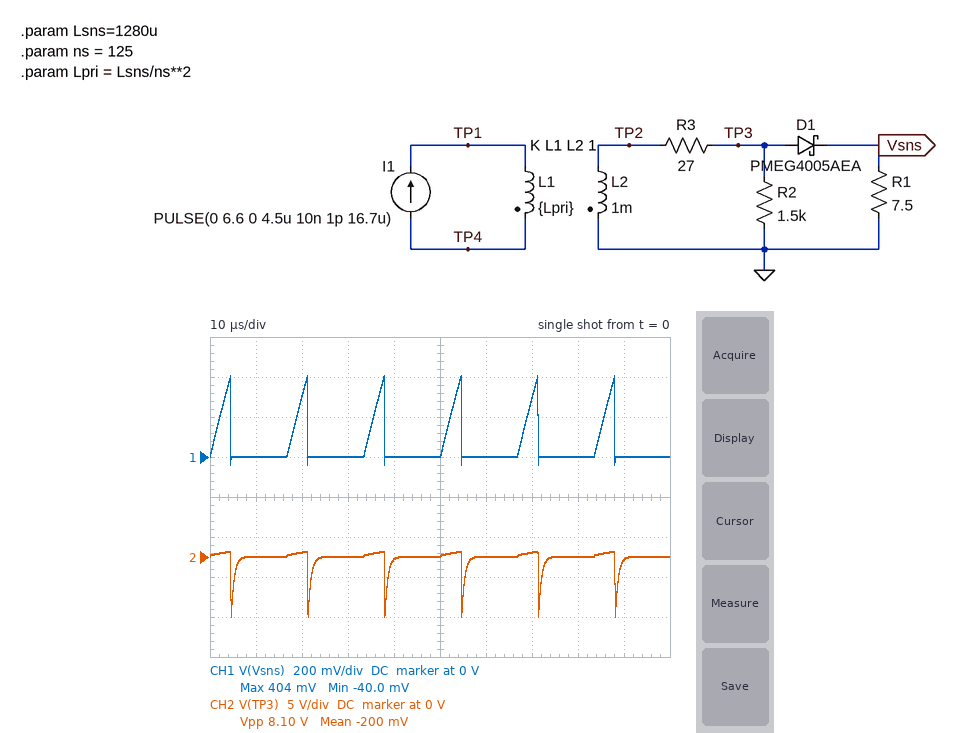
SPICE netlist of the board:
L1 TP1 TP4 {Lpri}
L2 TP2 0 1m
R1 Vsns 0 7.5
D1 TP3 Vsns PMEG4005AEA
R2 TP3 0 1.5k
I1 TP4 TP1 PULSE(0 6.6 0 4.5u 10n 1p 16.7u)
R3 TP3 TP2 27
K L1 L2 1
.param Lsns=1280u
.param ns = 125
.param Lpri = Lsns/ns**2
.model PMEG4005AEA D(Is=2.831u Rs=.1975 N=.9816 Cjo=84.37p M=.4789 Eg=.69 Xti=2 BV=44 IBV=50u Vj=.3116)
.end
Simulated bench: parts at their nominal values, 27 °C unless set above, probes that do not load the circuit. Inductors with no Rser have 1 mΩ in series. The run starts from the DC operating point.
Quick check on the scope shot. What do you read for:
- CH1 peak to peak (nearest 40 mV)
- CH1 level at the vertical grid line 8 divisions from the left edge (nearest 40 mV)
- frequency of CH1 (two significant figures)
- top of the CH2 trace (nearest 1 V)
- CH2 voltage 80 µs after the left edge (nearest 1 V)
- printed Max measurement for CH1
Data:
440 mV
0 V
60 kHz
1 V
0 V
404 mV
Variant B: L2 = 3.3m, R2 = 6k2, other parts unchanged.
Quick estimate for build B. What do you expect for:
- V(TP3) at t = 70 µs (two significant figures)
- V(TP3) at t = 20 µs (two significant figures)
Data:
400 mV
410 mV
